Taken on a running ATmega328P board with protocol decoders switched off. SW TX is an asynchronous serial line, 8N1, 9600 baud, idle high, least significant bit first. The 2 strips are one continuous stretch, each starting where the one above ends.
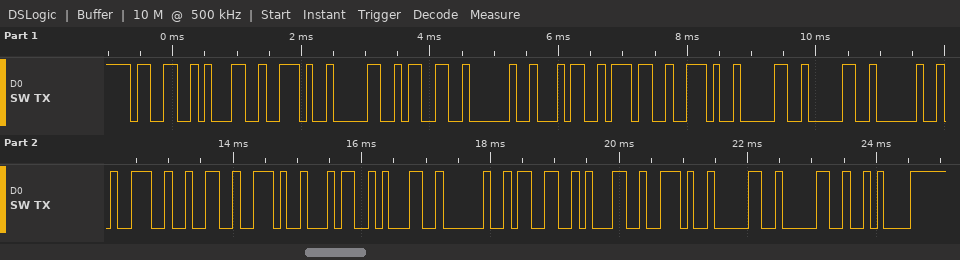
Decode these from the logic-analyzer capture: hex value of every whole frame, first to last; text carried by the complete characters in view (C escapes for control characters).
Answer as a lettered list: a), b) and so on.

a) 33 31 2E 30 33 20 34 37 2E 30 30 20 39 32 2E 34 31 20 33 31 2E 30 30 0A
b) "31.03 47.00 92.41 31.00\n"
